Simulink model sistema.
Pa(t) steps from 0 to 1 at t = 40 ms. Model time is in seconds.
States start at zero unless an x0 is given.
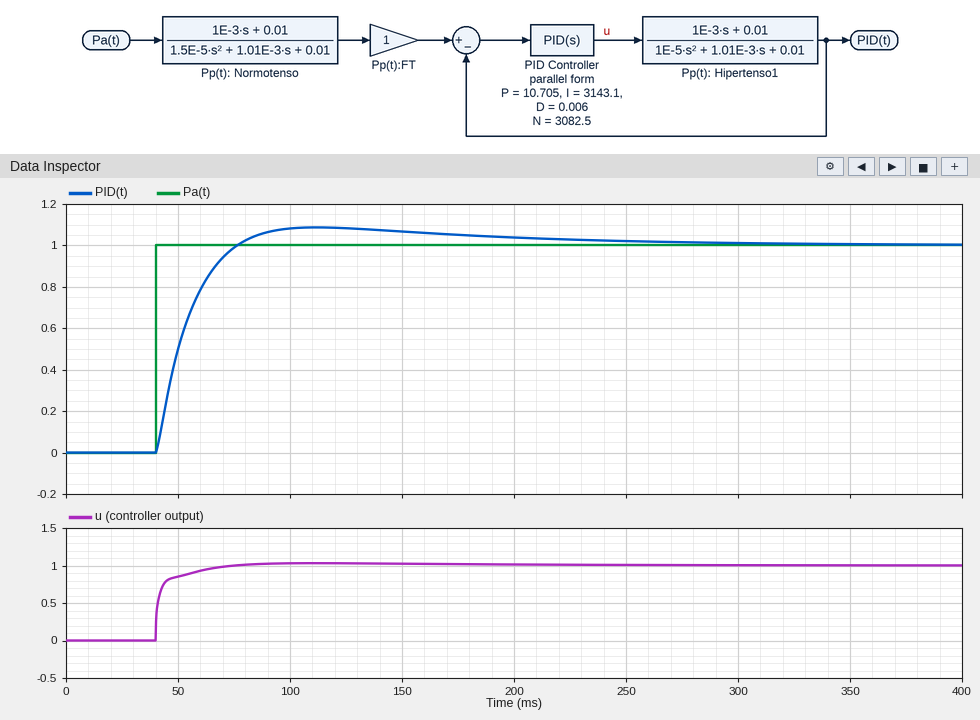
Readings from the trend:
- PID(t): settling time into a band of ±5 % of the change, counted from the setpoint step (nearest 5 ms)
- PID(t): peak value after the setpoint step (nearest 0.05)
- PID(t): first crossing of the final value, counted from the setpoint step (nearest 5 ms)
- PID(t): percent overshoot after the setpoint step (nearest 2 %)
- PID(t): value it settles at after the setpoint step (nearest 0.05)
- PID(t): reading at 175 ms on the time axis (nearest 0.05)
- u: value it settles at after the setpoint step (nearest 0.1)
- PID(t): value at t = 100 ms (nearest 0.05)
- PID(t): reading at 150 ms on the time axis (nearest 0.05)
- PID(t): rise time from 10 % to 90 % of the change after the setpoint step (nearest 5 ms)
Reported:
135 ms
1.10
35 ms
8 %
1.00
1.05
1.0
1.10
1.05
25 ms
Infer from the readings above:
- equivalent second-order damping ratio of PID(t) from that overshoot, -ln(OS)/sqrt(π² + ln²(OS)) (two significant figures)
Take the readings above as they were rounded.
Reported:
0.63
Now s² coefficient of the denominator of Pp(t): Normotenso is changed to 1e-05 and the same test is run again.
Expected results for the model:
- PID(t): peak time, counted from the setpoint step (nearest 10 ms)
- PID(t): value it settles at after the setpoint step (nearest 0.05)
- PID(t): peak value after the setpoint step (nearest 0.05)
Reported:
50 ms
1.00
1.05
